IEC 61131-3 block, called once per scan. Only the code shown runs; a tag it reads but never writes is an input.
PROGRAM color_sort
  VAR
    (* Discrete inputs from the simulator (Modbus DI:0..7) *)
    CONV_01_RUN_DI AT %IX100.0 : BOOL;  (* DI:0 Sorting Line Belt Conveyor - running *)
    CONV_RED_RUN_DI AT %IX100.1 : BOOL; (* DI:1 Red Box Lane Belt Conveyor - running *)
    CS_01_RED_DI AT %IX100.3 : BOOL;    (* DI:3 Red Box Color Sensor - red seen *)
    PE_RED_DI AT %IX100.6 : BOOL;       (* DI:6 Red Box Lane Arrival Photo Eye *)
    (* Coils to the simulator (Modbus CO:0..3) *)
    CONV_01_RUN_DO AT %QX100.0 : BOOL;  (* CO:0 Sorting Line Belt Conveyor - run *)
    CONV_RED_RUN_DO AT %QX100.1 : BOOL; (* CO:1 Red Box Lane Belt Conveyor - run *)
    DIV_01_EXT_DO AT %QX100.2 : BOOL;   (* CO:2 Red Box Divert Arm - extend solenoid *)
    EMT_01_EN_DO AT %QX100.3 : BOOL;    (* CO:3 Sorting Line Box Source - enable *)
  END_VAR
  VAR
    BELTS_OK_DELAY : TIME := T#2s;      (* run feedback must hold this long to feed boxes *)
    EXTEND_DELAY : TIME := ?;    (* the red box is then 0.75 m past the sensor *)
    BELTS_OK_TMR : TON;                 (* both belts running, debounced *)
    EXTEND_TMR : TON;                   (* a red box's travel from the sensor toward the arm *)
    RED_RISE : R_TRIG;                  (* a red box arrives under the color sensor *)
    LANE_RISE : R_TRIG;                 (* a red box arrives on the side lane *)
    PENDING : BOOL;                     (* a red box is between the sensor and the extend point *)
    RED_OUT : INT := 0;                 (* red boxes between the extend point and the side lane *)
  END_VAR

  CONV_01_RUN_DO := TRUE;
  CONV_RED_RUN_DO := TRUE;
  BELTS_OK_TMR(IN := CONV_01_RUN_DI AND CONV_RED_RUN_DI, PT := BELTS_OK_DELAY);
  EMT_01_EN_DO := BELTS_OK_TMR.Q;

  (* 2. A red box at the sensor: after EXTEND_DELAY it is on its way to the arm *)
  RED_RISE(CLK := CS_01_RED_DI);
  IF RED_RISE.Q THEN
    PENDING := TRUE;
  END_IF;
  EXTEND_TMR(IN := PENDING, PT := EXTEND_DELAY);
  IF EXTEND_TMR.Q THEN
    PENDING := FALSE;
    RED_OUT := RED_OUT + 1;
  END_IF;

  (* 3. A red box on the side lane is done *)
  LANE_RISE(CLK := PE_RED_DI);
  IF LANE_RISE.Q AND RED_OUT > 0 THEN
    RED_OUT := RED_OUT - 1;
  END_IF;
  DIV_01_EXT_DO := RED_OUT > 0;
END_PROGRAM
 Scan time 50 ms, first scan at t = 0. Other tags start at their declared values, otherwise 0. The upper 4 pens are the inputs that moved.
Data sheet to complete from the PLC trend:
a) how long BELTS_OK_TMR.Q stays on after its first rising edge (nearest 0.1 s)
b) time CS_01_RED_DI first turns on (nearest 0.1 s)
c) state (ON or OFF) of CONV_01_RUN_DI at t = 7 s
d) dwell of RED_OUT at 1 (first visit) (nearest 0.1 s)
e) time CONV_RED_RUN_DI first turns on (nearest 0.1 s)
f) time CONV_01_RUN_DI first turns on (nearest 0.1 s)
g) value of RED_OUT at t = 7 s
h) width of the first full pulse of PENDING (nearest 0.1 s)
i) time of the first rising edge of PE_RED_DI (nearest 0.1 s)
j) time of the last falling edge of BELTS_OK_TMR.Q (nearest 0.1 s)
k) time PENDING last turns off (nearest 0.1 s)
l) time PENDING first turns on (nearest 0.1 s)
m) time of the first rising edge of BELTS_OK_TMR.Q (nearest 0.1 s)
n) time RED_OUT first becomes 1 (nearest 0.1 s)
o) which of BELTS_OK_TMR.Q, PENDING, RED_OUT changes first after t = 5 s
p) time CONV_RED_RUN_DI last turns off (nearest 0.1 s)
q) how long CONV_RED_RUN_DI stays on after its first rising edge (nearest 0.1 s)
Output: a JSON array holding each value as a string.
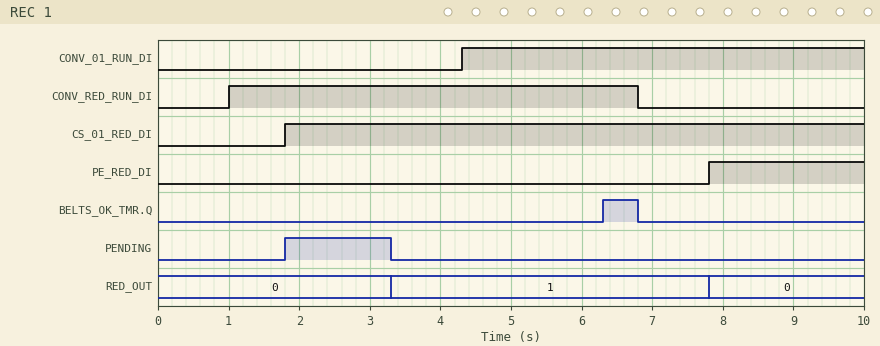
["0.5 s", "1.8 s", "ON", "4.5 s", "1.0 s", "4.3 s", "1", "1.5 s", "7.8 s", "6.8 s", "3.3 s", "1.8 s", "6.3 s", "3.3 s", "BELTS_OK_TMR.Q", "6.8 s", "5.8 s"]
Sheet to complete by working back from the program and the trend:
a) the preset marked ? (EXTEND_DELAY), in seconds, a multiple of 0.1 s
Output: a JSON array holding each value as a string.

["1.5 s"]
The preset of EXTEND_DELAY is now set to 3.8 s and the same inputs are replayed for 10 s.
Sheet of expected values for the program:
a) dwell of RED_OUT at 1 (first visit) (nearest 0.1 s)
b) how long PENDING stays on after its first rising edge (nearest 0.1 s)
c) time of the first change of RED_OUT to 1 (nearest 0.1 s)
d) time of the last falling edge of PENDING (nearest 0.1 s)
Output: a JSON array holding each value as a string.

["2.2 s", "3.8 s", "5.6 s", "5.6 s"]
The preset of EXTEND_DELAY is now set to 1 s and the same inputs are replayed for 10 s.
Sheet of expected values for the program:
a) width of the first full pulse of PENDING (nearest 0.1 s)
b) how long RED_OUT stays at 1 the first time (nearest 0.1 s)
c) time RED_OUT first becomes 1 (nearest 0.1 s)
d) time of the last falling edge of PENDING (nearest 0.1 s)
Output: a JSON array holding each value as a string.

["1.0 s", "5.0 s", "2.8 s", "2.8 s"]
